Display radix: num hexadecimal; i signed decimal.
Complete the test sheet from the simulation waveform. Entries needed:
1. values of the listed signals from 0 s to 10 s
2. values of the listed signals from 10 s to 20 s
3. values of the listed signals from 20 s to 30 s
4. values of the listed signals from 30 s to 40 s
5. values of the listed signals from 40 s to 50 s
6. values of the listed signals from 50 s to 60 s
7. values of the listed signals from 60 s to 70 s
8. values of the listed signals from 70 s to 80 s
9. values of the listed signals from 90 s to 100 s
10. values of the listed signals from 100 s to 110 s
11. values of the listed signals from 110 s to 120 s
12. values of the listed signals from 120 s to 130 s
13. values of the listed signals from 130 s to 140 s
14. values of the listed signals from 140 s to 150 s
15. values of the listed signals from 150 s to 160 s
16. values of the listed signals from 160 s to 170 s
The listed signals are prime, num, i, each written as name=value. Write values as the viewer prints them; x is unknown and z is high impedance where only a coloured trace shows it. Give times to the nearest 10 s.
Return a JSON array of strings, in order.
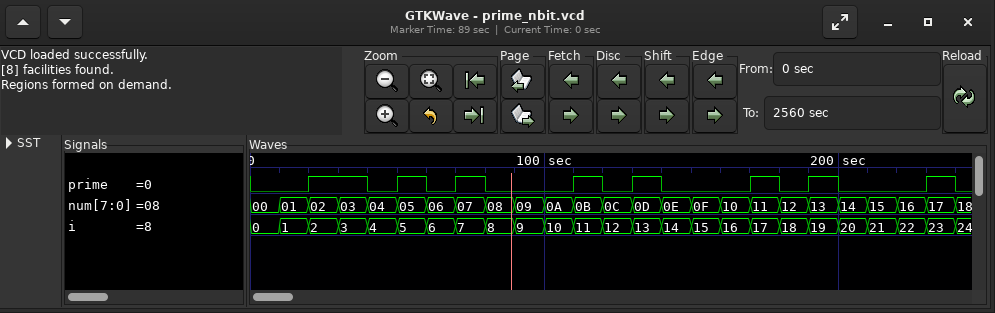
["prime=0, num=00, i=0", "prime=0, num=01, i=1", "prime=1, num=02, i=2", "prime=1, num=03, i=3", "prime=0, num=04, i=4", "prime=1, num=05, i=5", "prime=0, num=06, i=6", "prime=1, num=07, i=7", "prime=0, num=09, i=9", "prime=0, num=0A, i=10", "prime=1, num=0B, i=11", "prime=0, num=0C, i=12", "prime=1, num=0D, i=13", "prime=0, num=0E, i=14", "prime=0, num=0F, i=15", "prime=0, num=10, i=16"]
